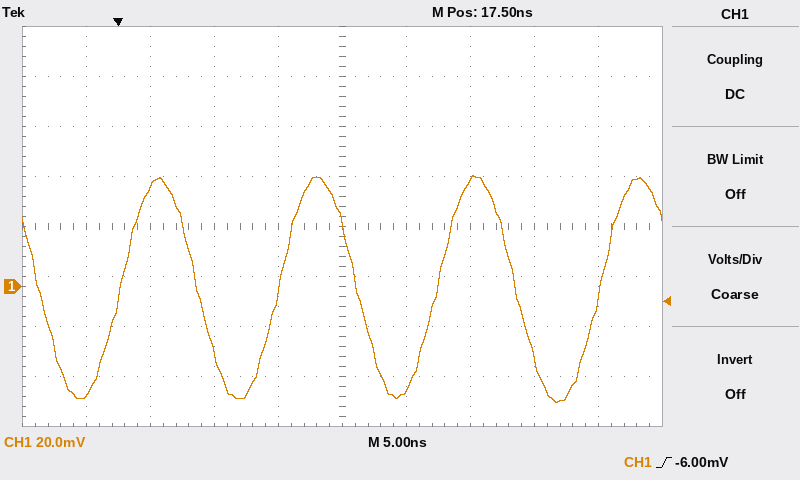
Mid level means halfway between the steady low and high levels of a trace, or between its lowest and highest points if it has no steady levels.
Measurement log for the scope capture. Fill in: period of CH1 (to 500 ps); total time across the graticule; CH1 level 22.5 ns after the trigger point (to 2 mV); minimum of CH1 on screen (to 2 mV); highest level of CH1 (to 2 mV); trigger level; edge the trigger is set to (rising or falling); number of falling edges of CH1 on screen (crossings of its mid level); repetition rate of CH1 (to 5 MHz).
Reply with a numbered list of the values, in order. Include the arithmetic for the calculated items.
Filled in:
1. 12.5 ns
2. 50 ns
3. -42 mV
4. -46 mV
5. 44 mV
6. -6.00 mV
7. rising
8. 4
9. 1 / 12.5 ns ≈ 80 MHz
